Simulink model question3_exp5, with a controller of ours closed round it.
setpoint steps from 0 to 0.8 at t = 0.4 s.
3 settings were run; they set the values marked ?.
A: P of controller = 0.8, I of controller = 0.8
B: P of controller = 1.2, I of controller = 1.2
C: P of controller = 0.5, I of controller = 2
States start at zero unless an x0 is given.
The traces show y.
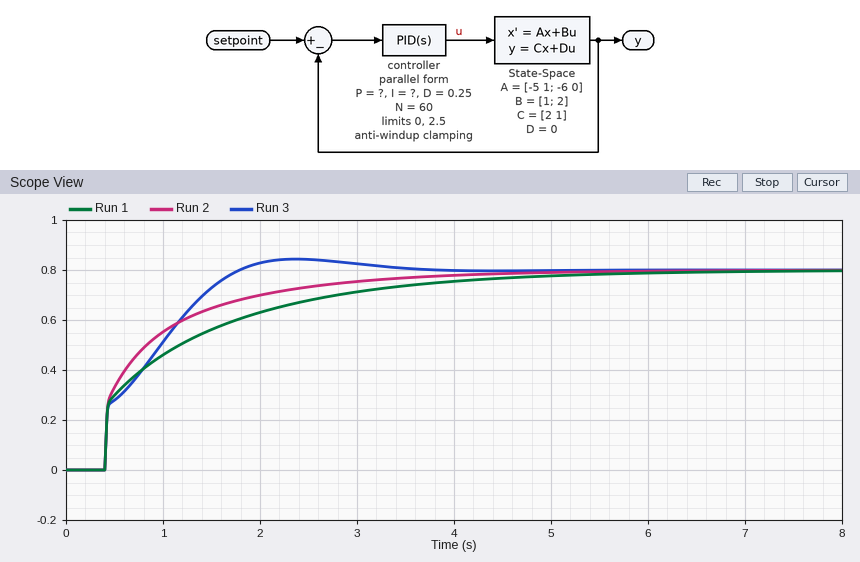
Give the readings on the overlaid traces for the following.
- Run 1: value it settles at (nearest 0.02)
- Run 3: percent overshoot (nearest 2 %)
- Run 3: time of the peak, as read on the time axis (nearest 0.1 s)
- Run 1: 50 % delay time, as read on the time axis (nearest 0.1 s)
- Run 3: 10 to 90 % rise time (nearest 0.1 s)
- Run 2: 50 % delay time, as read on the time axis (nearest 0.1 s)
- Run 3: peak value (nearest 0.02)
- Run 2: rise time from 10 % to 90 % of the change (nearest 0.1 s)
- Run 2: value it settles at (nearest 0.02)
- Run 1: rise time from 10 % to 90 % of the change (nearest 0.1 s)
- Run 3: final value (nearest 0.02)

0.80
6 %
2.4 s
0.8 s
1.1 s
0.6 s
0.84
1.9 s
0.80
2.7 s
0.80
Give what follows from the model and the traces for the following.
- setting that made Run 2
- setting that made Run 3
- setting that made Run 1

B
C
A
